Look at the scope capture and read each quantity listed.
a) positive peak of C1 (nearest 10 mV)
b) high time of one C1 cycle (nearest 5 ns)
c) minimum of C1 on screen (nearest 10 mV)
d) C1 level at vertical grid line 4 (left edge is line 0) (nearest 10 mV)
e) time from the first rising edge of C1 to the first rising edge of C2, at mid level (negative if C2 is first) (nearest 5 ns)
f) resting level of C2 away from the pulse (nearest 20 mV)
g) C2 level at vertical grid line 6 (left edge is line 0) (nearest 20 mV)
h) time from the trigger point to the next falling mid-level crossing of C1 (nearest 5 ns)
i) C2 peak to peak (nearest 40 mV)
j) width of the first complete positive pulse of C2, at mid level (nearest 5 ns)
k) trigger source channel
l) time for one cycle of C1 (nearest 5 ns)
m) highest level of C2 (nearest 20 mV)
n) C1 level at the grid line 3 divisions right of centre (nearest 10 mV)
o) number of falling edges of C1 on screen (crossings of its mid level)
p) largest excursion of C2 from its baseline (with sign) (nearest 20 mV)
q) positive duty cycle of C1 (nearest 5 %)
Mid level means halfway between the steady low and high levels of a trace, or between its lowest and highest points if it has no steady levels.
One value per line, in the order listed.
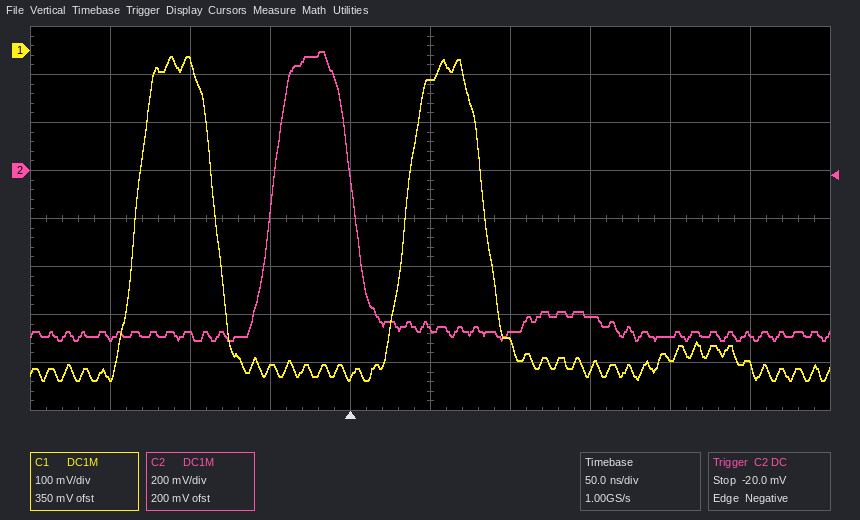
-10 mV
50 ns
-690 mV
-680 mV
+85 ns
-680 mV
-680 mV
85 ns
1.20 V
50 ns
C2
170 ns
500 mV
-640 mV
2
+1.18 V
30 %
